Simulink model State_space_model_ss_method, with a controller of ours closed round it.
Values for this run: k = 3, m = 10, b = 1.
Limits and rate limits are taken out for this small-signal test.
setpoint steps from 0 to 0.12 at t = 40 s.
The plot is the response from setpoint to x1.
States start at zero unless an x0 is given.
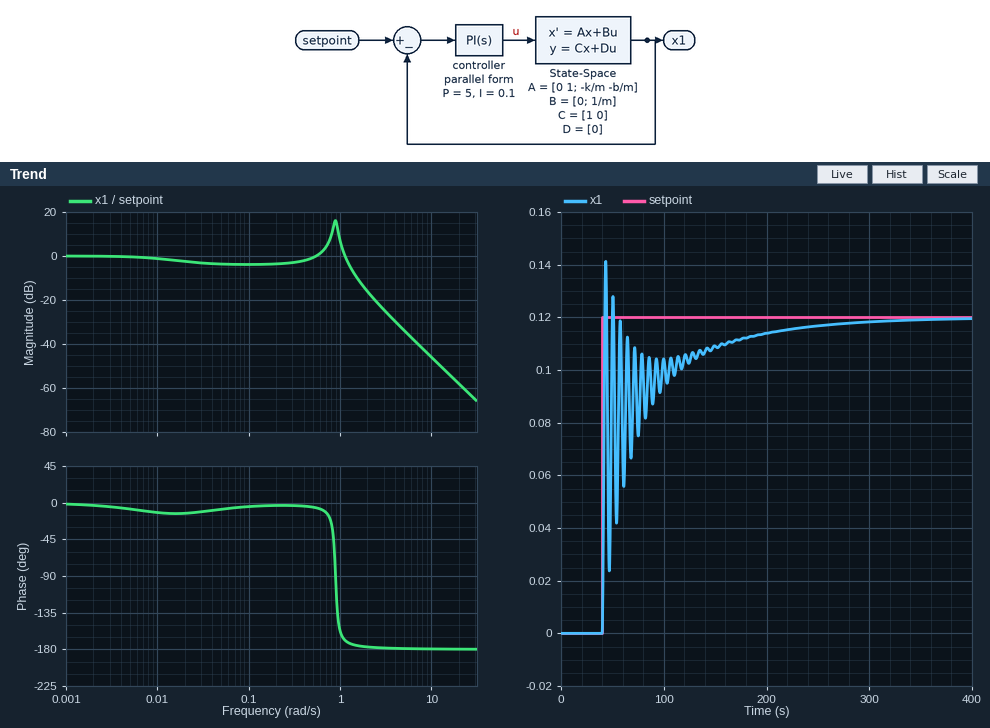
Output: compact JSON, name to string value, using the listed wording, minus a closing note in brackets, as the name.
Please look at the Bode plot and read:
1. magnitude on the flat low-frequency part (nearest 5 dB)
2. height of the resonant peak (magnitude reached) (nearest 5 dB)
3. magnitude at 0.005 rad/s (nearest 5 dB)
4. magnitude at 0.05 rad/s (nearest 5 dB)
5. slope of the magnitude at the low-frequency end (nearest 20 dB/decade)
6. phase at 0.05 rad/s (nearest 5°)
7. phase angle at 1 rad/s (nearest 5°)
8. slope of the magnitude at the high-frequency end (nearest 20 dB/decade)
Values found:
{"magnitude on the flat low-frequency part": "0 dB", "height of the resonant peak (magnitude reached)": "15 dB", "magnitude at 0.005 rad/s": "0 dB", "magnitude at 0.05 rad/s": "-5 dB", "slope of the magnitude at the low-frequency end": "0 dB/decade", "phase at 0.05 rad/s": "-10°", "phase angle at 1 rad/s": "-155°", "slope of the magnitude at the high-frequency end": "-40 dB/decade"}
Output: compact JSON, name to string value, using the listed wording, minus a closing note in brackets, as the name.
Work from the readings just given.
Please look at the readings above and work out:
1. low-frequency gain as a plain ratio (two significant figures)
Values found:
{"low-frequency gain as a plain ratio": "1.0"}
